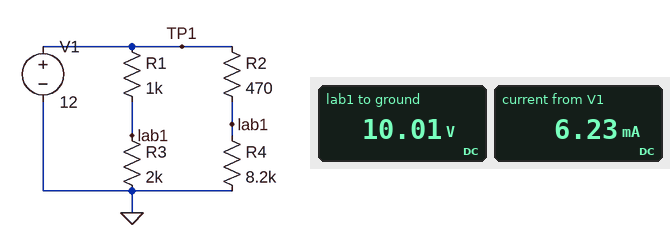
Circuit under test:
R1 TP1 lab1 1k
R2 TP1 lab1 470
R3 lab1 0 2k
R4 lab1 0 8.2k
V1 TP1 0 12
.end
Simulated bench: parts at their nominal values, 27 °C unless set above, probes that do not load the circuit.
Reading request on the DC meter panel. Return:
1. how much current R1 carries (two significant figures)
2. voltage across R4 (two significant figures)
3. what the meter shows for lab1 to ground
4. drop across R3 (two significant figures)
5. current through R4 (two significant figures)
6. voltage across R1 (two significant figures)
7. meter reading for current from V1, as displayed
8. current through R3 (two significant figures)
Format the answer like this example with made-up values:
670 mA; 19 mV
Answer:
2.0 mA; 10 V; 10.01 V; 10 V; 1.2 mA; 2.0 V; 6.23 mA; 5.0 mA
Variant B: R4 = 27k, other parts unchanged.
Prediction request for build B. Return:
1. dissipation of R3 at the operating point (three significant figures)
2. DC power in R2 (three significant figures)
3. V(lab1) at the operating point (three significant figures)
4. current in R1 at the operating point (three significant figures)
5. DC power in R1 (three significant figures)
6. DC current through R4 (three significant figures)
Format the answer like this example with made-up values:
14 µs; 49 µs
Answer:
52.4 mW; 6.58 mW; 10.2 V; 1.76 mA; 3.09 mW; 379 µA
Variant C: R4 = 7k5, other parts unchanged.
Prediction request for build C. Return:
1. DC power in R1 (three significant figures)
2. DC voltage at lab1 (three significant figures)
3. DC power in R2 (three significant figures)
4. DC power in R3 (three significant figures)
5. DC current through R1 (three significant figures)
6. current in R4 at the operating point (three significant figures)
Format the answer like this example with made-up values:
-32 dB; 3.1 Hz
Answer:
4.08 mW; 9.98 V; 8.69 mW; 49.8 mW; 2.02 mA; 1.33 mA
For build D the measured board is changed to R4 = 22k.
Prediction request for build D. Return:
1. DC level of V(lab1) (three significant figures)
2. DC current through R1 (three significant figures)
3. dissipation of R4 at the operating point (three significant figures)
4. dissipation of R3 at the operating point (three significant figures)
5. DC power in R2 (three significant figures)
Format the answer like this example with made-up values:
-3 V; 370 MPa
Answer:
10.2 V; 1.78 mA; 4.75 mW; 52.2 mW; 6.76 mW
